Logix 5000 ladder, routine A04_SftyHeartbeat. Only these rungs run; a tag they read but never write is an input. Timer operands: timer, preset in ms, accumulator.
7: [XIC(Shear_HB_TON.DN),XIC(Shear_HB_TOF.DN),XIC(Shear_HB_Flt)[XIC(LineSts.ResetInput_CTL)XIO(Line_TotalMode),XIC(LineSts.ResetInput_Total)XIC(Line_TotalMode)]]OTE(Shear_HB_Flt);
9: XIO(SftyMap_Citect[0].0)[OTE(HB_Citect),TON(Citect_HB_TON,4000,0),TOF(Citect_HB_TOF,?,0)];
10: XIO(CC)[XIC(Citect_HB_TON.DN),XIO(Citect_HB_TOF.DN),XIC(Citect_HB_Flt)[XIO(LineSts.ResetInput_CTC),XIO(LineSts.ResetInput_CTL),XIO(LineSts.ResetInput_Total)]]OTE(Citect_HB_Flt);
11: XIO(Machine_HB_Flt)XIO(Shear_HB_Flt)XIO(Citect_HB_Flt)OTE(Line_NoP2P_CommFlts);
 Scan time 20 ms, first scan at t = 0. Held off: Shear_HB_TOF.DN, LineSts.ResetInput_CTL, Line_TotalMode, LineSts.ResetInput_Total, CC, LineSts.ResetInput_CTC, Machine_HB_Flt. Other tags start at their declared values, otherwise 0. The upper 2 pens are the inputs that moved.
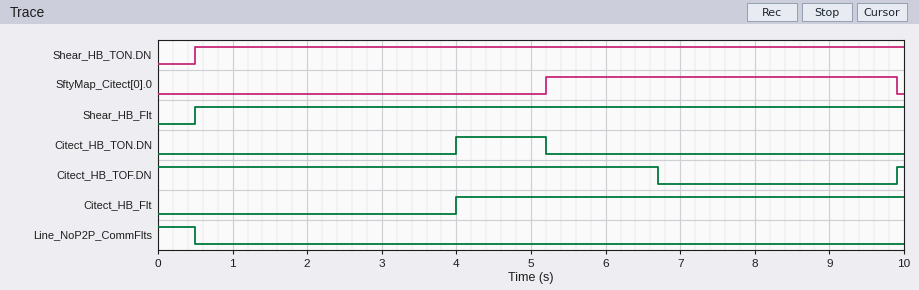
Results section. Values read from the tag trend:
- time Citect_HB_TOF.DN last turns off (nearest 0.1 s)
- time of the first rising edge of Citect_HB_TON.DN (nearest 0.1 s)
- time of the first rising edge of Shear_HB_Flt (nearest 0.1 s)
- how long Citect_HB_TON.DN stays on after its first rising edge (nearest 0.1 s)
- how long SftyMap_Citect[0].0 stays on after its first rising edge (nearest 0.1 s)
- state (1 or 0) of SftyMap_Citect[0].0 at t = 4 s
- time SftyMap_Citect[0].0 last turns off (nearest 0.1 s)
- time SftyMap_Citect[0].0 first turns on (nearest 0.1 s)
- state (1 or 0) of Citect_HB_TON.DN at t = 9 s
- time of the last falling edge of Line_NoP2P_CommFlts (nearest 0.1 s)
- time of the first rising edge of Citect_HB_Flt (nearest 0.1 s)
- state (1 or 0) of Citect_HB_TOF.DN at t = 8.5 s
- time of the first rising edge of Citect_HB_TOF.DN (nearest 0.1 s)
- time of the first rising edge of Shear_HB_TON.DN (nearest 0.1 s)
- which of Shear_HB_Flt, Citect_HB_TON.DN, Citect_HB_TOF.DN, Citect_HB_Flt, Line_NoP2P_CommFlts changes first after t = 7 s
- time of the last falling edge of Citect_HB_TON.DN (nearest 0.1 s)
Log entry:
6.7 s
4.0 s
0.5 s
1.2 s
4.7 s
0
9.9 s
5.2 s
0
0.5 s
4.0 s
0
9.9 s
0.5 s
Citect_HB_TOF.DN
5.2 s
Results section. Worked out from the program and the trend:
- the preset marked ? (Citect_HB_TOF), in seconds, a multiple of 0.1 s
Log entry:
1.5 s
